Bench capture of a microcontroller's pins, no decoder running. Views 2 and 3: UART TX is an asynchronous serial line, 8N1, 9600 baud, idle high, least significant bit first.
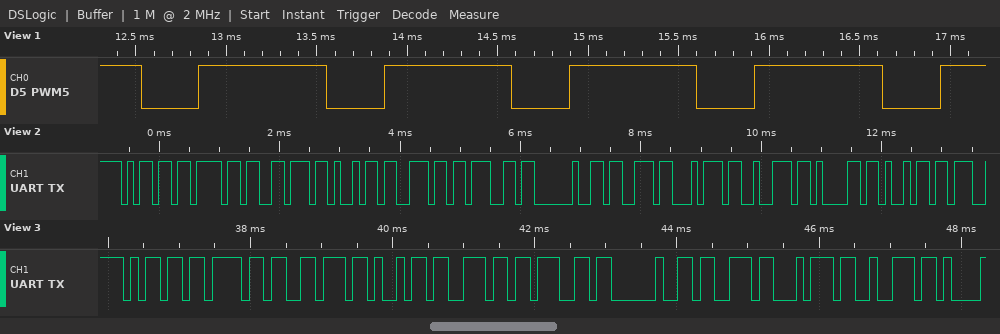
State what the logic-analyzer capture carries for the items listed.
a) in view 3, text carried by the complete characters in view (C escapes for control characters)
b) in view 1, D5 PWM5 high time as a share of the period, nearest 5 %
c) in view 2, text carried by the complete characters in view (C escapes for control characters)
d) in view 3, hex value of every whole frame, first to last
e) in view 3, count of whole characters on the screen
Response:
"moving str"
70 %
"moving strai"
6D 6F 76 69 6E 67 20 73 74 72
10
